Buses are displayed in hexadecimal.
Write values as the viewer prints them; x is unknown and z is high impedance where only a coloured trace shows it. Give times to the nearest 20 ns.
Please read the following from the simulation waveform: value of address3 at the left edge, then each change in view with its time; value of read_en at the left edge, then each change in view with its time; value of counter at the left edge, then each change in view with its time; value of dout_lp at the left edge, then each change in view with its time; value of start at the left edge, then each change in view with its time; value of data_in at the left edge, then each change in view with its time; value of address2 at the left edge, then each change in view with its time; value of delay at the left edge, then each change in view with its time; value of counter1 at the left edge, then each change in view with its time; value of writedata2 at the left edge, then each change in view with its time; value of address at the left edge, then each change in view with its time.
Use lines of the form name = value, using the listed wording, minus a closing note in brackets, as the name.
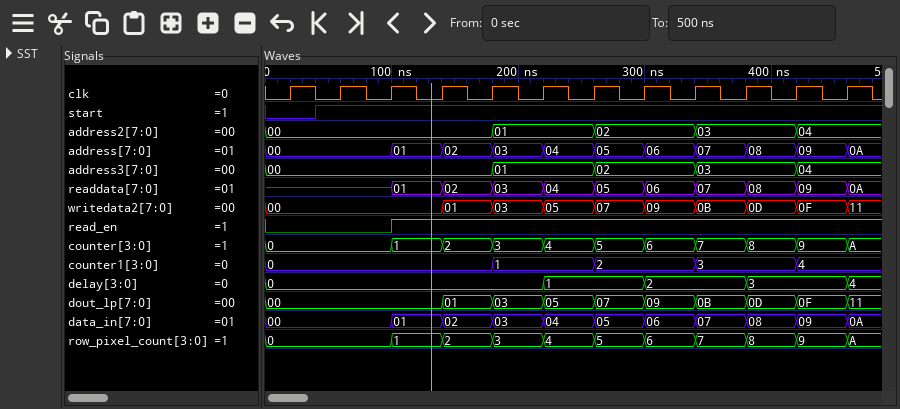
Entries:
value of address3 at the left edge, then each change in view with its time = 00, 01 at 180 ns, 02 at 260 ns, 03 at 340 ns, 04 at 420 ns
value of read_en at the left edge, then each change in view with its time = 0, 1 at 100 ns
value of counter at the left edge, then each change in view with its time = 0, 1 at 100 ns, 2 at 140 ns, 3 at 180 ns, 4 at 220 ns, 5 at 260 ns, 6 at 300 ns, 7 at 340 ns, 8 at 380 ns, 9 at 420 ns, A at 460 ns
value of dout_lp at the left edge, then each change in view with its time = 00, 01 at 140 ns, 03 at 180 ns, 05 at 220 ns, 07 at 260 ns, 09 at 300 ns, 0B at 340 ns, 0D at 380 ns, 0F at 420 ns, 11 at 460 ns
value of start at the left edge, then each change in view with its time = 0, 1 at 40 ns
value of data_in at the left edge, then each change in view with its time = 00, 01 at 100 ns, 02 at 140 ns, 03 at 180 ns, 04 at 220 ns, 05 at 260 ns, 06 at 300 ns, 07 at 340 ns, 08 at 380 ns, 09 at 420 ns, 0A at 460 ns
value of address2 at the left edge, then each change in view with its time = 00, 01 at 180 ns, 02 at 260 ns, 03 at 340 ns, 04 at 420 ns
value of delay at the left edge, then each change in view with its time = 0, 1 at 220 ns, 2 at 300 ns, 3 at 380 ns, 4 at 460 ns
value of counter1 at the left edge, then each change in view with its time = 0, 1 at 180 ns, 2 at 260 ns, 3 at 340 ns, 4 at 420 ns
value of writedata2 at the left edge, then each change in view with its time = 00, 01 at 140 ns, 03 at 180 ns, 05 at 220 ns, 07 at 260 ns, 09 at 300 ns, 0B at 340 ns, 0D at 380 ns, 0F at 420 ns, 11 at 460 ns
value of address at the left edge, then each change in view with its time = 00, 01 at 100 ns, 02 at 140 ns, 03 at 180 ns, 04 at 220 ns, 05 at 260 ns, 06 at 300 ns, 07 at 340 ns, 08 at 380 ns, 09 at 420 ns, 0A at 460 ns
